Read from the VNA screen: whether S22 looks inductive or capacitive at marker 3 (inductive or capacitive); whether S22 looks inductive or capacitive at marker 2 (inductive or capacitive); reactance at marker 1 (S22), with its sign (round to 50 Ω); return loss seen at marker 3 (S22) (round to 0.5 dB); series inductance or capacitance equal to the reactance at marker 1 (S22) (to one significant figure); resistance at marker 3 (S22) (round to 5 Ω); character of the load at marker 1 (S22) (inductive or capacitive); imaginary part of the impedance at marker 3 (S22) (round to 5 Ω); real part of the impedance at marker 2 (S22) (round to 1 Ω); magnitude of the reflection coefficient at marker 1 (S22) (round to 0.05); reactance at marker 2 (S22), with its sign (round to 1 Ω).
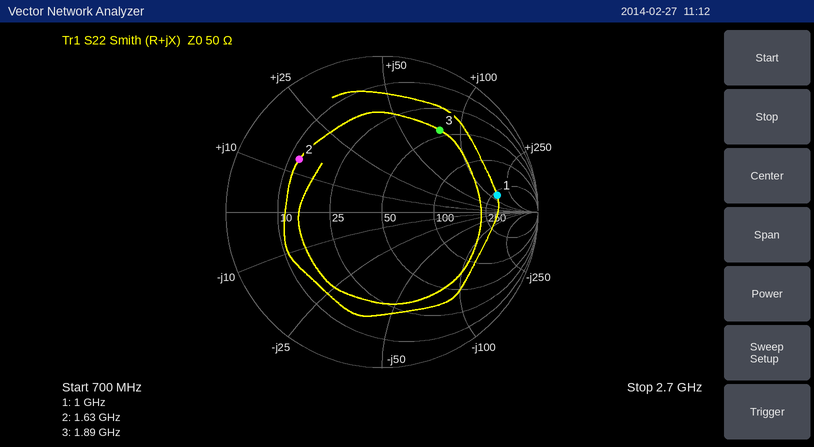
inductive
inductive
+150 Ω
4.0 dB
20 nH
45 Ω
inductive
+80 Ω
12 Ω
0.75
+14 Ω
